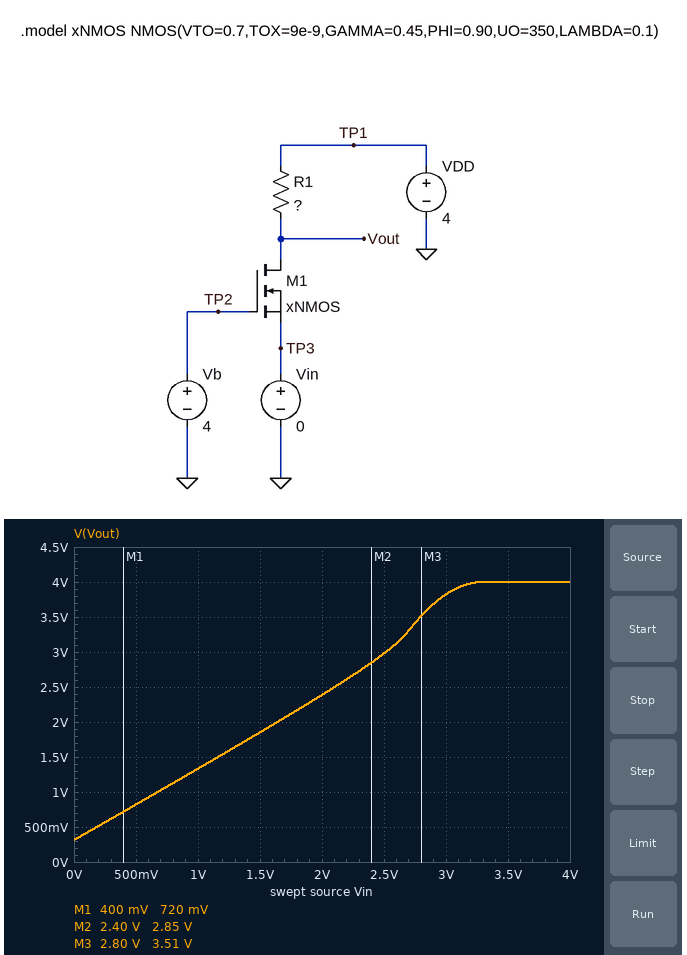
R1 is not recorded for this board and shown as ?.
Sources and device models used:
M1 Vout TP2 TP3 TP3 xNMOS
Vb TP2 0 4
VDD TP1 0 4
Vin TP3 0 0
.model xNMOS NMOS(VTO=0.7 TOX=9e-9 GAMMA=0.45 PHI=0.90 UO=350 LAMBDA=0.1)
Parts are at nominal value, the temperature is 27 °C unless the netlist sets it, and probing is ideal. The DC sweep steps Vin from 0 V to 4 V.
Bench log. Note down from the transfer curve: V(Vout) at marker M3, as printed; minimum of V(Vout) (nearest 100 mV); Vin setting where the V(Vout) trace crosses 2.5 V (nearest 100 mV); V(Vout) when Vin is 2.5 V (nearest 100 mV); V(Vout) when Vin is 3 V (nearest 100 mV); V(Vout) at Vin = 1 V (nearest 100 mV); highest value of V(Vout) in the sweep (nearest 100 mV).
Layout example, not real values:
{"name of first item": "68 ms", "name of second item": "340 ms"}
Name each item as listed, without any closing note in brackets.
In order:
{"V(Vout) at marker M3, as printed": "3.51 V", "minimum of V(Vout)": "300 mV", "Vin setting where the V(Vout) trace crosses 2.5 V": "2.1 V", "V(Vout) when Vin is 2.5 V": "3.0 V", "V(Vout) when Vin is 3 V": "3.8 V", "V(Vout) at Vin = 1 V": "1.3 V", "highest value of V(Vout) in the sweep": "4.0 V"}
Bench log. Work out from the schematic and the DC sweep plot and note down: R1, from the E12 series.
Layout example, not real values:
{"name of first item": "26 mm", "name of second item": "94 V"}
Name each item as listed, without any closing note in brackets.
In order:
{"R1, from the E12 series": "27 kΩ"}
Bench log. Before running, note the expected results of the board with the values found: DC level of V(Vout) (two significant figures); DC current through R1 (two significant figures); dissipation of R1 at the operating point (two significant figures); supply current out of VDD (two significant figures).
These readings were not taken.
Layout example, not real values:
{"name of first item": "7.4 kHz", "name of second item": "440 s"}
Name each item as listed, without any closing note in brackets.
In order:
{"DC level of V(Vout)": "310 mV", "DC current through R1": "140 µA", "dissipation of R1 at the operating point": "500 µW", "supply current out of VDD": "140 µA"}
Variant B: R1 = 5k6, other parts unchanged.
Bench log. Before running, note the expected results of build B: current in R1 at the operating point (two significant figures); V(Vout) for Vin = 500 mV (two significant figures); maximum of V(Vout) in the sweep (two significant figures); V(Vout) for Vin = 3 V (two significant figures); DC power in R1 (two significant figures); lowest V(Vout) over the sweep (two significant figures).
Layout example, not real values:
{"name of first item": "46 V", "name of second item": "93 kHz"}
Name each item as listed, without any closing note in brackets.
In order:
{"current in R1 at the operating point": "500 µA", "V(Vout) for Vin = 500 mV": "1.7 V", "maximum of V(Vout) in the sweep": "4.0 V", "V(Vout) for Vin = 3 V": "4.0 V", "DC power in R1": "1.4 mW", "lowest V(Vout) over the sweep": "1.2 V"}
